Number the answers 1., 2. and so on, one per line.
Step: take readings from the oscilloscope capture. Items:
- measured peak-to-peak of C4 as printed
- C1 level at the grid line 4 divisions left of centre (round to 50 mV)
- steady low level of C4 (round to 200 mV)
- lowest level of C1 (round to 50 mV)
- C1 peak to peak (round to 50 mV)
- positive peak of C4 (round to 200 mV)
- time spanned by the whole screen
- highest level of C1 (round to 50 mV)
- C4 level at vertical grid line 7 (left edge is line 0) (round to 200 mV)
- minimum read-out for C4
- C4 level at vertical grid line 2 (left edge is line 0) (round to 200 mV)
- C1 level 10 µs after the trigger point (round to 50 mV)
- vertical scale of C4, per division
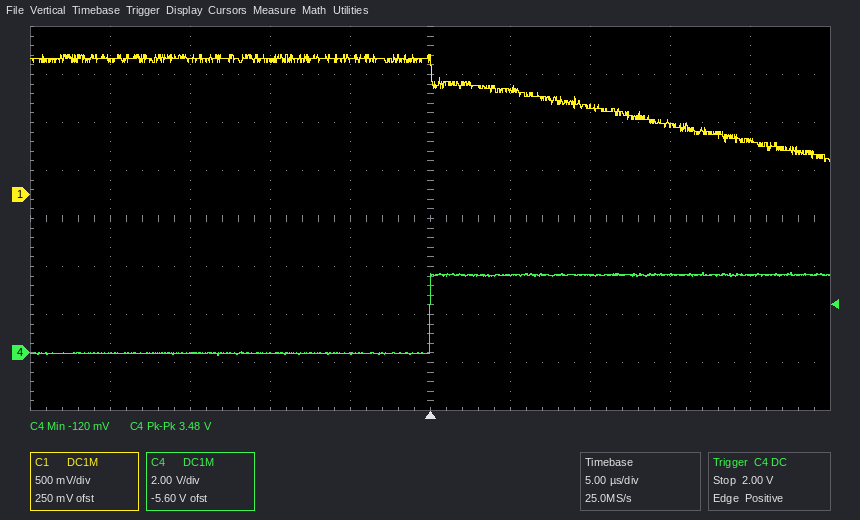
1. 3.48 V
2. 1.40 V
3. 0.0 V
4. 350 mV
5. 1.10 V
6. 3.4 V
7. 50 µs
8. 1.45 V
9. 3.2 V
10. -120 mV
11. 0.0 V
12. 900 mV
13. 2 V
